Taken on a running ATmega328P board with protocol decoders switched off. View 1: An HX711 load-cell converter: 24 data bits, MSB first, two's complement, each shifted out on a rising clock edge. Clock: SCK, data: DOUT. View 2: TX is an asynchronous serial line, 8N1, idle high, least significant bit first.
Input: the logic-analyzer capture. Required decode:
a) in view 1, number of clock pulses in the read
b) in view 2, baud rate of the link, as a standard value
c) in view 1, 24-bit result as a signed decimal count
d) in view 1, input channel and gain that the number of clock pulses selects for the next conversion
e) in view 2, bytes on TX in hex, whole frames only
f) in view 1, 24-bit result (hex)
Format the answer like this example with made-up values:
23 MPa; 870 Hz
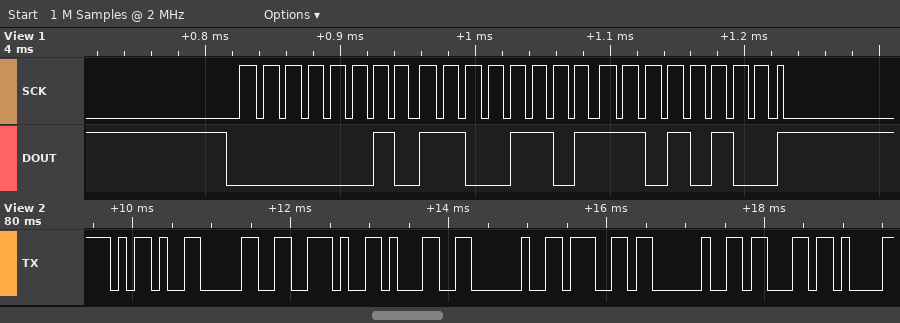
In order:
25; 9600 baud; 183764; channel A, gain 128; 0x2D 0x30 0x2E 0x31 0x20 0x67 0x20 0x63; 0x02CDD4
